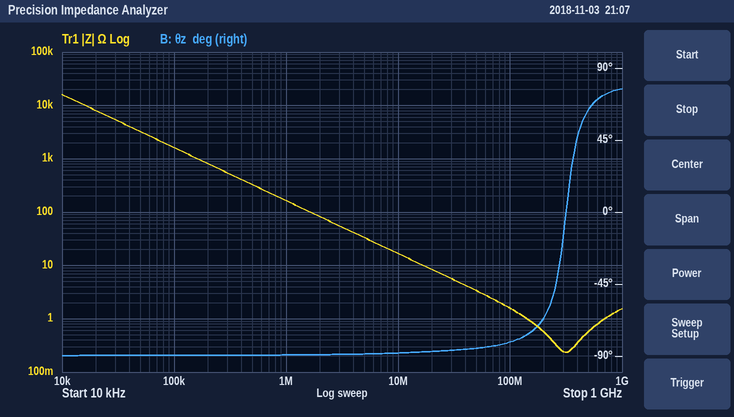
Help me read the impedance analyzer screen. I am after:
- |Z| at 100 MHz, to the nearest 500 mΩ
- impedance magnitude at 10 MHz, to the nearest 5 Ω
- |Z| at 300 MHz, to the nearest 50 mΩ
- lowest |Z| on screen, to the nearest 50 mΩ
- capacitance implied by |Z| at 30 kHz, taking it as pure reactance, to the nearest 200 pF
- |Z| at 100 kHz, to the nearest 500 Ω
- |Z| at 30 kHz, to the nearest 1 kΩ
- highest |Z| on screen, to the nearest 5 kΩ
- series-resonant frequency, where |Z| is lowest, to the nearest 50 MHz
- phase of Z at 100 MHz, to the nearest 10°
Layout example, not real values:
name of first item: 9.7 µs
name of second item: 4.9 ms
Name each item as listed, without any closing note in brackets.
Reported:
|Z| at 100 MHz, to the nearest 500 mΩ: 1.5 Ω
impedance magnitude at 10 MHz, to the nearest 5 Ω: 15 Ω
|Z| at 300 MHz, to the nearest 50 mΩ: 250 mΩ
lowest |Z| on screen, to the nearest 50 mΩ: 250 mΩ
capacitance implied by |Z| at 30 kHz, taking it as pure reactance, to the nearest 200 pF: 1.0 nF
|Z| at 100 kHz, to the nearest 500 Ω: 1.5 kΩ
|Z| at 30 kHz, to the nearest 1 kΩ: 5 kΩ
highest |Z| on screen, to the nearest 5 kΩ: 15 kΩ
series-resonant frequency, where |Z| is lowest, to the nearest 50 MHz: 300 MHz
phase of Z at 100 MHz, to the nearest 10°: -80°
